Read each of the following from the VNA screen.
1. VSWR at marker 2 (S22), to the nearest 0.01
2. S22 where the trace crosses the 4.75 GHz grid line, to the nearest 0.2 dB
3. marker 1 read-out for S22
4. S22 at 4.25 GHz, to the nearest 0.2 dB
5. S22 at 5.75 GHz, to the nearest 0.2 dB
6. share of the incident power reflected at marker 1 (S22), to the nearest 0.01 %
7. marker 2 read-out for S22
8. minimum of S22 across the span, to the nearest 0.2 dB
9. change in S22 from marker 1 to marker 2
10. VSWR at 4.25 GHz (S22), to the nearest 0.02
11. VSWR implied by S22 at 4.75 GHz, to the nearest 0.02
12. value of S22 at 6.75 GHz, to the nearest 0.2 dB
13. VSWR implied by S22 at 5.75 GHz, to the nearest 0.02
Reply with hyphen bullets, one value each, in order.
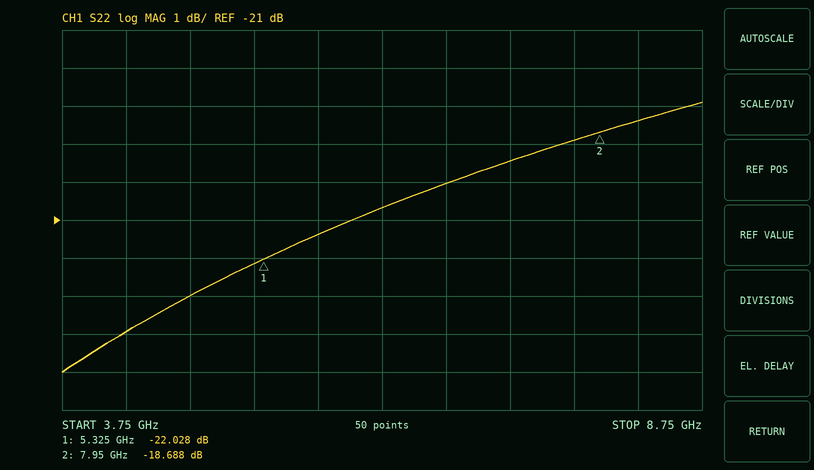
- 1.26
- -23.0 dB
- -22.028 dB
- -24.0 dB
- -21.4 dB
- 0.63 %
- -18.688 dB
- -25.0 dB
- 3.340 dB
- 1.14
- 1.16
- -20.0 dB
- 1.18
